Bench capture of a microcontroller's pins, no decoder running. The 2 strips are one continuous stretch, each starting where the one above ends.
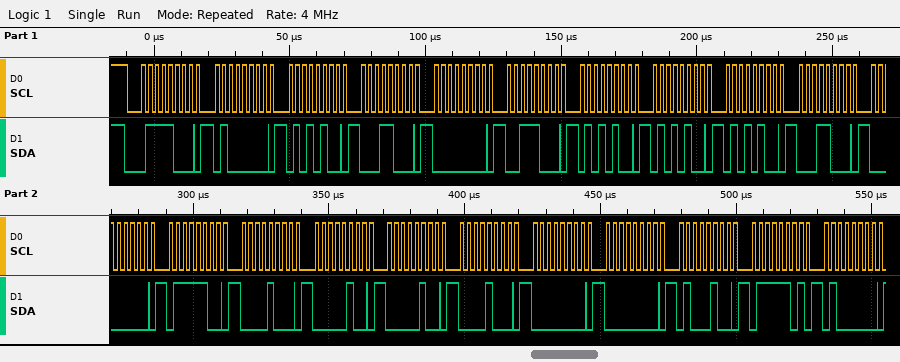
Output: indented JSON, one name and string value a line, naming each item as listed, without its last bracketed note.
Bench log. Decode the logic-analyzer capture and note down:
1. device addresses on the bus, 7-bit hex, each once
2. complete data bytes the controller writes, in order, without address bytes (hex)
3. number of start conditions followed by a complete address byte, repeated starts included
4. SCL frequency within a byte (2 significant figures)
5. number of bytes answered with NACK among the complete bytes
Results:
{
  "device addresses on the bus, 7-bit hex, each once": "0x3C",
  "complete data bytes the controller writes, in order, without address bytes": "40 54 18 00 38 54 54 54 18 00 7C 08 04 04 08 00 00 44 7D 40",
  "number of start conditions followed by a complete address byte, repeated starts included": "1",
  "SCL frequency within a byte": "400 kHz",
  "number of bytes answered with NACK among the complete bytes": "0"
}
